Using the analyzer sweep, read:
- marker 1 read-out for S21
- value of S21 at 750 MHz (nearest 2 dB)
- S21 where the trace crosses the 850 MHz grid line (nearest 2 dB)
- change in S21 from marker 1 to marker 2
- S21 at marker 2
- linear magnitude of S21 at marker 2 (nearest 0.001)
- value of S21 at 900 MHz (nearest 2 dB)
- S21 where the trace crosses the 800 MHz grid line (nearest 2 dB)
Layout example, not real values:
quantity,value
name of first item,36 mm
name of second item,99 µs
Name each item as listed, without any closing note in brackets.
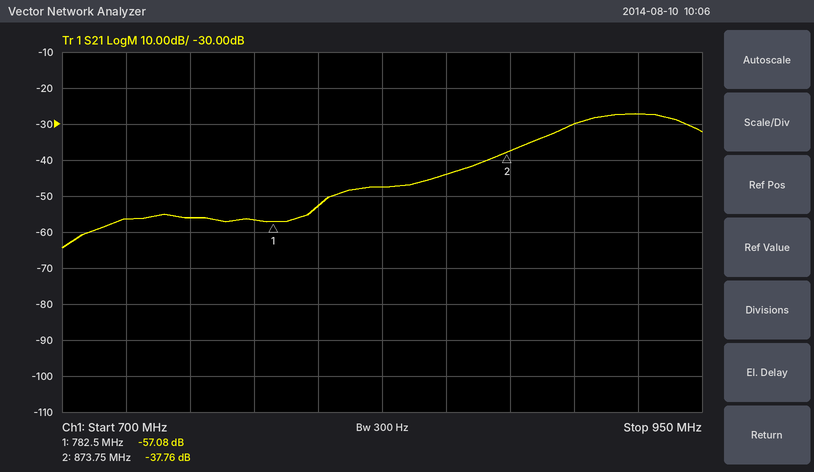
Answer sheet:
quantity,value
marker 1 read-out for S21,-57.08 dB
value of S21 at 750 MHz,-56 dB
S21 where the trace crosses the 850 MHz grid line,-44 dB
change in S21 from marker 1 to marker 2,19.32 dB
S21 at marker 2,-37.76 dB
linear magnitude of S21 at marker 2,0.013
value of S21 at 900 MHz,-30 dB
S21 where the trace crosses the 800 MHz grid line,-52 dB
